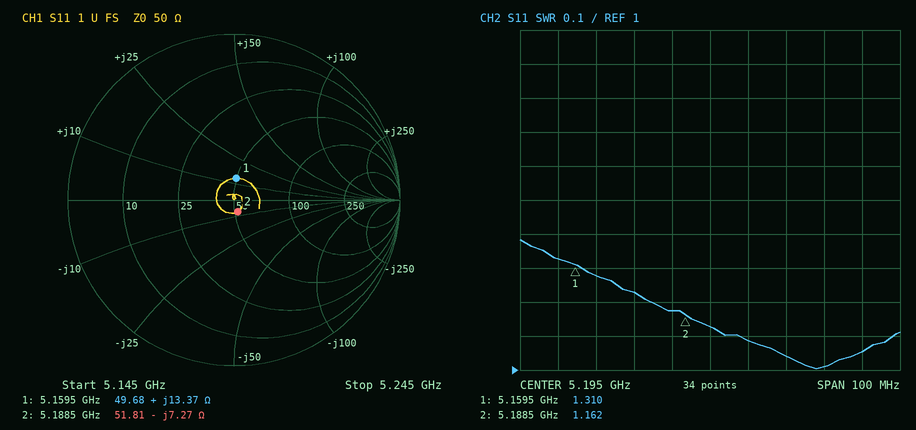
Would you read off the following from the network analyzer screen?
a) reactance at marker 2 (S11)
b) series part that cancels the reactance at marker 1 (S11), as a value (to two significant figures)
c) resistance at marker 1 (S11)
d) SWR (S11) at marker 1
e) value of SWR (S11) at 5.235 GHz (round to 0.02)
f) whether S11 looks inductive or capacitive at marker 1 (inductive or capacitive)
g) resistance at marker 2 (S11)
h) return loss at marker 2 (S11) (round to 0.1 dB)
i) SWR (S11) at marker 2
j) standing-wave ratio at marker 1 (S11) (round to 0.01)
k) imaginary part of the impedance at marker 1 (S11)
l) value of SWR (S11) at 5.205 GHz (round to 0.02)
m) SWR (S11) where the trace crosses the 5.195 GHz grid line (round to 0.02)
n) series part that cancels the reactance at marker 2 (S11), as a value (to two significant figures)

-7.27 Ω
2.3 pF
49.68 Ω
1.310
1.06
inductive
51.81 Ω
22.7 dB
1.162
1.31
+13.37 Ω
1.08
1.12
220 pH
